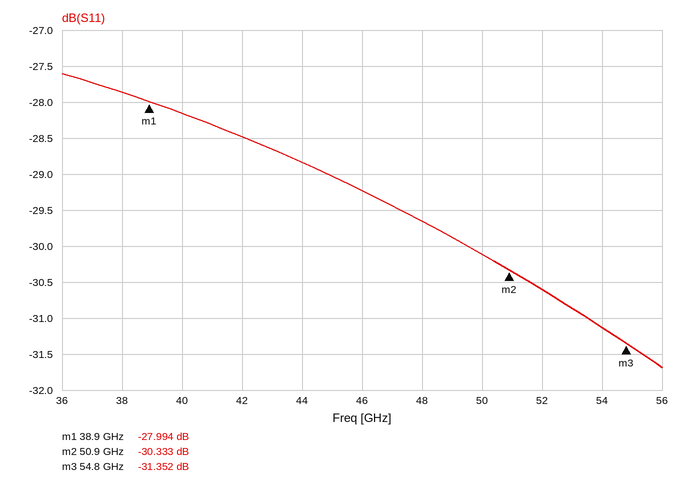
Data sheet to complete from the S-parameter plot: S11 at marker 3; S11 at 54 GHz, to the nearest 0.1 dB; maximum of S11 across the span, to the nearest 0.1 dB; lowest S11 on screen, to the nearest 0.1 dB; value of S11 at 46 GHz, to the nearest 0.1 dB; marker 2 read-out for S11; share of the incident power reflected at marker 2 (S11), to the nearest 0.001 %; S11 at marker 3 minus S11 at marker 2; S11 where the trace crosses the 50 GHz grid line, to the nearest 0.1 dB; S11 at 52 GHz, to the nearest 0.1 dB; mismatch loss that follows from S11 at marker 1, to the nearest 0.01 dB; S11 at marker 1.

-31.352 dB
-31.1 dB
-27.6 dB
-31.7 dB
-29.2 dB
-30.333 dB
0.093 %
-1.019 dB
-30.1 dB
-30.6 dB
0.01 dB
-27.994 dB
